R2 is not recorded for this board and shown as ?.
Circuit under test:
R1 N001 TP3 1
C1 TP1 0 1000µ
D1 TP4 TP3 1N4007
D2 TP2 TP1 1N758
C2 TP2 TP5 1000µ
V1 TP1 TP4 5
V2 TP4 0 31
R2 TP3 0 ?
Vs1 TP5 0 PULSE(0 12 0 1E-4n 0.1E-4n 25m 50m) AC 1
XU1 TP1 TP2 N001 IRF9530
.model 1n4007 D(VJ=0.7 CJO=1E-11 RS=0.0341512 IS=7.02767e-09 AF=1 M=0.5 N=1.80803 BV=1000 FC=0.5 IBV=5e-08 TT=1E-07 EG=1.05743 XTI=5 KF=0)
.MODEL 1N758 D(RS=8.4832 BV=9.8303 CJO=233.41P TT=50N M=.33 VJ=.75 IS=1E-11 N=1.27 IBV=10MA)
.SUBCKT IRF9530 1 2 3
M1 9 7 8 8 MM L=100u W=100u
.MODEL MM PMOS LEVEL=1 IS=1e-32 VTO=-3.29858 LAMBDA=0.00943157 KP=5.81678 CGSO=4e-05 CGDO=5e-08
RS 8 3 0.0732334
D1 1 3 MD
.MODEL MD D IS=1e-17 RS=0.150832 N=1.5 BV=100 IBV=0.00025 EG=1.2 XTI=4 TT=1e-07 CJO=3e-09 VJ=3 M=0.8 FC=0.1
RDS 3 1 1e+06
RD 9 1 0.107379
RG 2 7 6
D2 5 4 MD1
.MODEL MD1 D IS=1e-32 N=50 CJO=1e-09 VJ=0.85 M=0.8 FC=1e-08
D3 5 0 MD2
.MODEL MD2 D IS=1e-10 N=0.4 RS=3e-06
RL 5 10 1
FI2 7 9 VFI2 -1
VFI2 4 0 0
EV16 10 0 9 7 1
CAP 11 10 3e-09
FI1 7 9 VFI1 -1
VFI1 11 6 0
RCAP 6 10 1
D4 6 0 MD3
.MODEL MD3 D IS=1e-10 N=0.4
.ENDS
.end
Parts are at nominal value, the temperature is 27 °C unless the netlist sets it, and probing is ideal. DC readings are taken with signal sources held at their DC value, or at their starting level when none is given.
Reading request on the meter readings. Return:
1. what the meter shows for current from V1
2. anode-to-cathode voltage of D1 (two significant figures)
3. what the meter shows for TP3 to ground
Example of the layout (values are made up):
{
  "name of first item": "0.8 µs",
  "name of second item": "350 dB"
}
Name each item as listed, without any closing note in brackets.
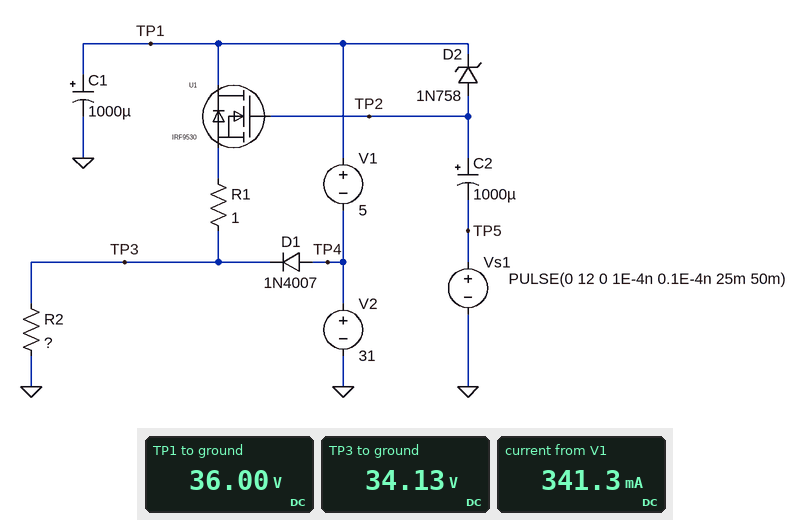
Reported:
{
  "what the meter shows for current from V1": "341.3 mA",
  "anode-to-cathode voltage of D1": "-3.1 V",
  "what the meter shows for TP3 to ground": "34.13 V"
}
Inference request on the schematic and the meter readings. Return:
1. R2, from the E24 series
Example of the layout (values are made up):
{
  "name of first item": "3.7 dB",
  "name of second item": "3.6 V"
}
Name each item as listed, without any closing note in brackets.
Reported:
{
  "R2, from the E24 series": "100 Ω"
}
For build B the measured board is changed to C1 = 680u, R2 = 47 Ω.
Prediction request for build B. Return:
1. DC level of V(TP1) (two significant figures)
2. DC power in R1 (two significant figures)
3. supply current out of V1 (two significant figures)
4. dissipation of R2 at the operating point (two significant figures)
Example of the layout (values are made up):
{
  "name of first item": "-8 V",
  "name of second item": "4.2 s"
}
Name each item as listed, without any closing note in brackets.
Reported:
{
  "DC level of V(TP1)": "36 V",
  "DC power in R1": "510 mW",
  "supply current out of V1": "720 mA",
  "dissipation of R2 at the operating point": "24 W"
}
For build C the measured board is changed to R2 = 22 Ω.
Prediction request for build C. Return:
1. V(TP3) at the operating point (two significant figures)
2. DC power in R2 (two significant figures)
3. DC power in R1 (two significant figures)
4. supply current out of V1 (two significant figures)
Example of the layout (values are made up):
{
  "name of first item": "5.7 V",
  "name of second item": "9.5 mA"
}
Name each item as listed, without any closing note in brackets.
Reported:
{
  "V(TP3) at the operating point": "33 V",
  "DC power in R2": "49 W",
  "DC power in R1": "2.2 W",
  "supply current out of V1": "1.5 A"
}
